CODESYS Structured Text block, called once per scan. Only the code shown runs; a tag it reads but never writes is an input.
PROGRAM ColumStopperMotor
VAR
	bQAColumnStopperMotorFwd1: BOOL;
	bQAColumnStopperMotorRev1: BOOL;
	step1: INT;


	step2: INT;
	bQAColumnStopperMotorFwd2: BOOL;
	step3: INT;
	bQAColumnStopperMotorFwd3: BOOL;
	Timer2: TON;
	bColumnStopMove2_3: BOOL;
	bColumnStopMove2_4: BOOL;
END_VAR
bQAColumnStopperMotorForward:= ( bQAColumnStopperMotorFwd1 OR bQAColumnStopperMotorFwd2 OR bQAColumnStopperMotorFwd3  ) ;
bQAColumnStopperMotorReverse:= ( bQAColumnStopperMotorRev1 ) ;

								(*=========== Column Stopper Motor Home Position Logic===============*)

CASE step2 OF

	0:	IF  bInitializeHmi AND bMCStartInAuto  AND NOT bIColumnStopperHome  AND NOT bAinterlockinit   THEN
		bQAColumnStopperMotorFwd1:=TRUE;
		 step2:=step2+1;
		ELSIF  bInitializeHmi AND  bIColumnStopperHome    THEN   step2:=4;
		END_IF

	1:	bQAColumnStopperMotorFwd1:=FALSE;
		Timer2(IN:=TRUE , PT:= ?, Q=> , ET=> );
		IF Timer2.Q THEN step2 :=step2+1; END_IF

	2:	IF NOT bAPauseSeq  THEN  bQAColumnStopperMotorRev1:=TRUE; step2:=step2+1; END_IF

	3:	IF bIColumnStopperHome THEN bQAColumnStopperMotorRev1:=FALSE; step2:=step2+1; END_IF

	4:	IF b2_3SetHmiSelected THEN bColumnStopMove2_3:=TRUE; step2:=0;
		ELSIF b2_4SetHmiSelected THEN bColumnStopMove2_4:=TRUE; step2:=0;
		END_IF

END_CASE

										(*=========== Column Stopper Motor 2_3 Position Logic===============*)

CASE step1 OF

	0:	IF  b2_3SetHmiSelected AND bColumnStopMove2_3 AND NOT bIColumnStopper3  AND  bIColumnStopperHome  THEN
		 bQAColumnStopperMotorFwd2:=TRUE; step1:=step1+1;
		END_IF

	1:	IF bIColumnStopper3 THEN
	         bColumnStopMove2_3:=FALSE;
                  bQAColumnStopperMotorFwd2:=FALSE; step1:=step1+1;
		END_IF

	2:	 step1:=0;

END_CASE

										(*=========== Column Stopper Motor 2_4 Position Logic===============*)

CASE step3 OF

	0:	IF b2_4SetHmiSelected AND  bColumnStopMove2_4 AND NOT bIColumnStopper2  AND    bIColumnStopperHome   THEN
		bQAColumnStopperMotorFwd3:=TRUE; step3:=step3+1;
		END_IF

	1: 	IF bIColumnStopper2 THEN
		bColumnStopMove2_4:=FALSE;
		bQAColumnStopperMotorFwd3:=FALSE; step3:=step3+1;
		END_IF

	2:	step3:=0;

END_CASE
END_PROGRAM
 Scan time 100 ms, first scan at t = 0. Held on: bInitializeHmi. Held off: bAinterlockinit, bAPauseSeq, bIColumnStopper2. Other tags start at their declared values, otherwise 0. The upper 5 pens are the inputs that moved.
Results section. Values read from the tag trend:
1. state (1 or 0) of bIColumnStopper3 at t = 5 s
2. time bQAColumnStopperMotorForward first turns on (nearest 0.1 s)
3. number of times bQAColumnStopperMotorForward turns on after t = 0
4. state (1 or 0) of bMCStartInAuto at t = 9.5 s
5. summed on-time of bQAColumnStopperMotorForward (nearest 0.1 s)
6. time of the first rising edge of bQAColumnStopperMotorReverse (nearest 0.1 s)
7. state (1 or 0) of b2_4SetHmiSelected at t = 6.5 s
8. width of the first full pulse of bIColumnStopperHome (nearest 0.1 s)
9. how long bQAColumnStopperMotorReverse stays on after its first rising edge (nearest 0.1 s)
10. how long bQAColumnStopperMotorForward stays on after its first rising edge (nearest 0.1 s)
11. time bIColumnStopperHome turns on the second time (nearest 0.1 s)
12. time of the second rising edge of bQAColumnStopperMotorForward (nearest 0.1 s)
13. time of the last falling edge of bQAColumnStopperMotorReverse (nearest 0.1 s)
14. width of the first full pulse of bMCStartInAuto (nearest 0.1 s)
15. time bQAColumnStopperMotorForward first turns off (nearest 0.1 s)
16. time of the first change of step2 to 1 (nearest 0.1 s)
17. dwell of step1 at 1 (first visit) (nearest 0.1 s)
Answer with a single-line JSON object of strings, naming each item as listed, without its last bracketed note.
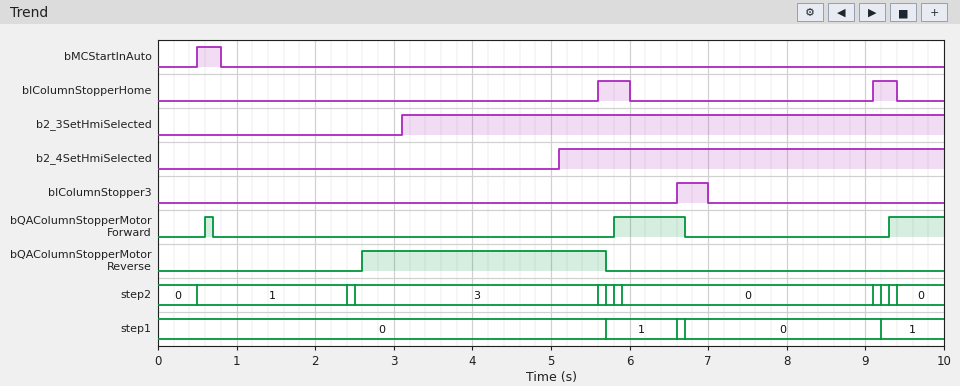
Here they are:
{"state (1 or 0) of bIColumnStopper3 at t = 5 s": "0", "time bQAColumnStopperMotorForward first turns on": "0.6 s", "number of times bQAColumnStopperMotorForward turns on after t = 0": "3", "state (1 or 0) of bMCStartInAuto at t = 9.5 s": "0", "summed on-time of bQAColumnStopperMotorForward": "1.7 s", "time of the first rising edge of bQAColumnStopperMotorReverse": "2.6 s", "state (1 or 0) of b2_4SetHmiSelected at t = 6.5 s": "1", "width of the first full pulse of bIColumnStopperHome": "0.4 s", "how long bQAColumnStopperMotorReverse stays on after its first rising edge": "3.1 s", "how long bQAColumnStopperMotorForward stays on after its first rising edge": "0.1 s", "time bIColumnStopperHome turns on the second time": "9.1 s", "time of the second rising edge of bQAColumnStopperMotorForward": "5.8 s", "time of the last falling edge of bQAColumnStopperMotorReverse": "5.7 s", "width of the first full pulse of bMCStartInAuto": "0.3 s", "time bQAColumnStopperMotorForward first turns off": "0.7 s", "time of the first change of step2 to 1": "0.5 s", "dwell of step1 at 1 (first visit)": "0.9 s"}
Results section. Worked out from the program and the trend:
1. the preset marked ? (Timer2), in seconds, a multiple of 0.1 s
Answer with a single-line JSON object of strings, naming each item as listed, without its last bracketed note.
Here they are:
{"the preset marked ? (Timer2), in seconds, a multiple of 0.1 s": "1.8 s"}
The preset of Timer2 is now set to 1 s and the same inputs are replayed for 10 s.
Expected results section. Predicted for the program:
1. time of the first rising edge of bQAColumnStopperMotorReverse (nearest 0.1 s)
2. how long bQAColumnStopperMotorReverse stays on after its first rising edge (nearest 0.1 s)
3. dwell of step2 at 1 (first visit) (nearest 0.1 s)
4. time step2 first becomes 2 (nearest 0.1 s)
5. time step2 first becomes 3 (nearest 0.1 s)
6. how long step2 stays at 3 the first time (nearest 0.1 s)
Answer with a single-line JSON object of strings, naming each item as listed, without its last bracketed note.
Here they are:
{"time of the first rising edge of bQAColumnStopperMotorReverse": "1.8 s", "how long bQAColumnStopperMotorReverse stays on after its first rising edge": "3.9 s", "dwell of step2 at 1 (first visit)": "1.1 s", "time step2 first becomes 2": "1.6 s", "time step2 first becomes 3": "1.7 s", "how long step2 stays at 3 the first time": "3.9 s"}
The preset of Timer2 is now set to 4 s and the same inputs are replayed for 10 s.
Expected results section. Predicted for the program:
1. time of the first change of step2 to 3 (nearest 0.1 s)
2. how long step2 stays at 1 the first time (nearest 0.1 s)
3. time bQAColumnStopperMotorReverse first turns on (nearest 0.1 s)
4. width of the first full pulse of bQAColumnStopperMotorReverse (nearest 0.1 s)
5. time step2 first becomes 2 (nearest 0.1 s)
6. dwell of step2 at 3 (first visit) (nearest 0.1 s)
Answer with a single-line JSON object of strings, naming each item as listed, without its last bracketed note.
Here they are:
{"time of the first change of step2 to 3": "4.7 s", "how long step2 stays at 1 the first time": "4.1 s", "time bQAColumnStopperMotorReverse first turns on": "4.8 s", "width of the first full pulse of bQAColumnStopperMotorReverse": "0.9 s", "time step2 first becomes 2": "4.6 s", "dwell of step2 at 3 (first visit)": "0.9 s"}
